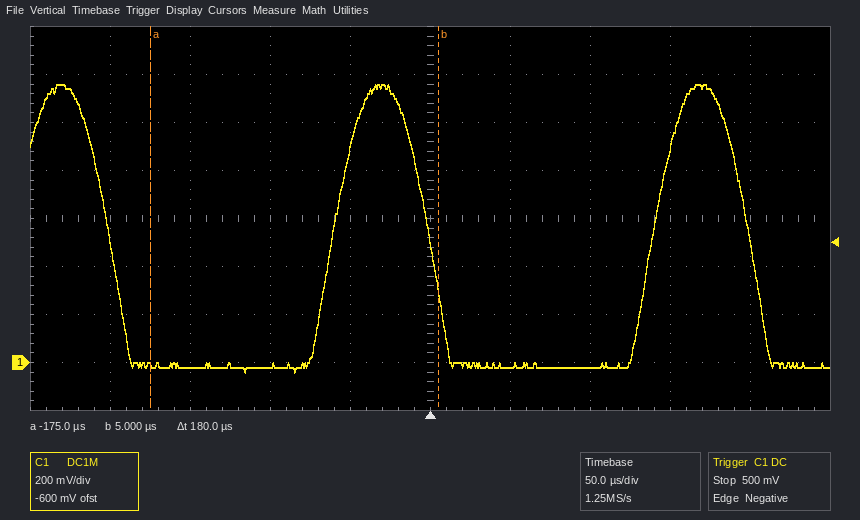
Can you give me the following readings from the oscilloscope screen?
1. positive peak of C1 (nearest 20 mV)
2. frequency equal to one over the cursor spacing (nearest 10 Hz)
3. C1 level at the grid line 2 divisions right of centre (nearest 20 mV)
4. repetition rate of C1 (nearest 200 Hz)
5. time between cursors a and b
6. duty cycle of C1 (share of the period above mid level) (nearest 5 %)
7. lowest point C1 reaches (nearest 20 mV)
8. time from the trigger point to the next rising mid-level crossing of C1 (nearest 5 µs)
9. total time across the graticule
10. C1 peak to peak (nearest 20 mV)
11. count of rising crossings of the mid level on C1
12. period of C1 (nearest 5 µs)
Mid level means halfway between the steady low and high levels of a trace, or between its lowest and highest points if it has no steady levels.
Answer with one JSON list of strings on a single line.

["1.16 V", "5.56 kHz", "-20 mV", "5.0 kHz", "180 µs", "30 %", "-40 mV", "140 µs", "500 µs", "1.20 V", "2", "200 µs"]
